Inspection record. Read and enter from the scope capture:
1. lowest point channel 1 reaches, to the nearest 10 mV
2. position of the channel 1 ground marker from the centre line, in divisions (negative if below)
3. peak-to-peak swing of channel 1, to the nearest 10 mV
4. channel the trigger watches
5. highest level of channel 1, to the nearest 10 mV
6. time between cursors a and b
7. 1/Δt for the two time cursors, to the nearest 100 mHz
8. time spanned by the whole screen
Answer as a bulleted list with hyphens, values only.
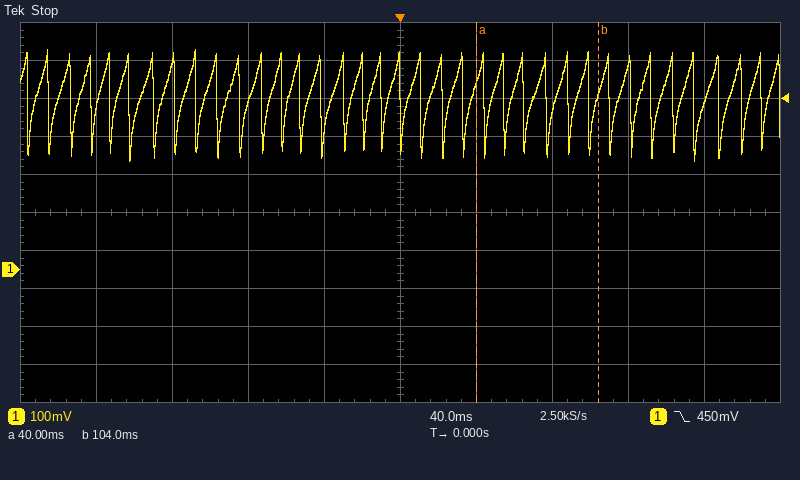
- 290 mV
- -1.5 div
- 290 mV
- channel 1
- 580 mV
- 64 ms
- 15.6 Hz
- 400 ms
